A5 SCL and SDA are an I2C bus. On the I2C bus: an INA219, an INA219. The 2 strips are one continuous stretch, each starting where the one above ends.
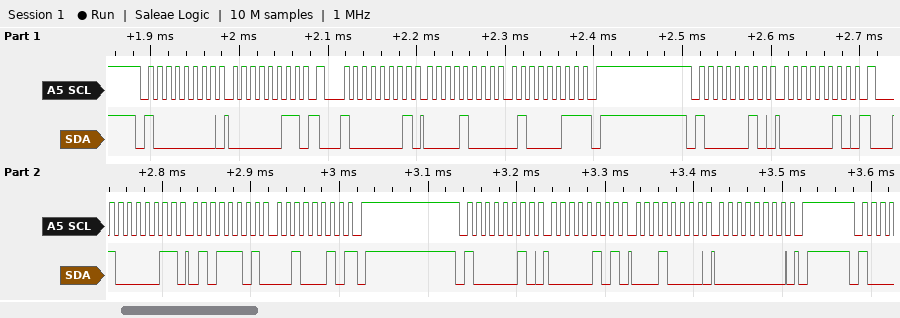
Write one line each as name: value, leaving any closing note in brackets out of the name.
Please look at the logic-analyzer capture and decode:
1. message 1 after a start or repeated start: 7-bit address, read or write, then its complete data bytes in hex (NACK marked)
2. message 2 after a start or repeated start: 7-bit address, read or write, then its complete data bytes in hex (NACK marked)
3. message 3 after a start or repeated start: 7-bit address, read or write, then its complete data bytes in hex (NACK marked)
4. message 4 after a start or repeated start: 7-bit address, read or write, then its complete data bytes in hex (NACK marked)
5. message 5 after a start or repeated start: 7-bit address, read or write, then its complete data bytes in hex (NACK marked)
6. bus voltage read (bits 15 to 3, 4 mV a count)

message 1 after a start or repeated start: 7-bit address, read or write, then its complete data bytes in hex: 0x40 write: 03
message 2 after a start or repeated start: 7-bit address, read or write, then its complete data bytes in hex: 0x40 read: 08 43 NACK
message 3 after a start or repeated start: 7-bit address, read or write, then its complete data bytes in hex: 0x41 write: 02
message 4 after a start or repeated start: 7-bit address, read or write, then its complete data bytes in hex: 0x41 read: 5D 22 NACK
message 5 after a start or repeated start: 7-bit address, read or write, then its complete data bytes in hex: 0x41 write: 05 10 00
bus voltage read: 11.920 V
